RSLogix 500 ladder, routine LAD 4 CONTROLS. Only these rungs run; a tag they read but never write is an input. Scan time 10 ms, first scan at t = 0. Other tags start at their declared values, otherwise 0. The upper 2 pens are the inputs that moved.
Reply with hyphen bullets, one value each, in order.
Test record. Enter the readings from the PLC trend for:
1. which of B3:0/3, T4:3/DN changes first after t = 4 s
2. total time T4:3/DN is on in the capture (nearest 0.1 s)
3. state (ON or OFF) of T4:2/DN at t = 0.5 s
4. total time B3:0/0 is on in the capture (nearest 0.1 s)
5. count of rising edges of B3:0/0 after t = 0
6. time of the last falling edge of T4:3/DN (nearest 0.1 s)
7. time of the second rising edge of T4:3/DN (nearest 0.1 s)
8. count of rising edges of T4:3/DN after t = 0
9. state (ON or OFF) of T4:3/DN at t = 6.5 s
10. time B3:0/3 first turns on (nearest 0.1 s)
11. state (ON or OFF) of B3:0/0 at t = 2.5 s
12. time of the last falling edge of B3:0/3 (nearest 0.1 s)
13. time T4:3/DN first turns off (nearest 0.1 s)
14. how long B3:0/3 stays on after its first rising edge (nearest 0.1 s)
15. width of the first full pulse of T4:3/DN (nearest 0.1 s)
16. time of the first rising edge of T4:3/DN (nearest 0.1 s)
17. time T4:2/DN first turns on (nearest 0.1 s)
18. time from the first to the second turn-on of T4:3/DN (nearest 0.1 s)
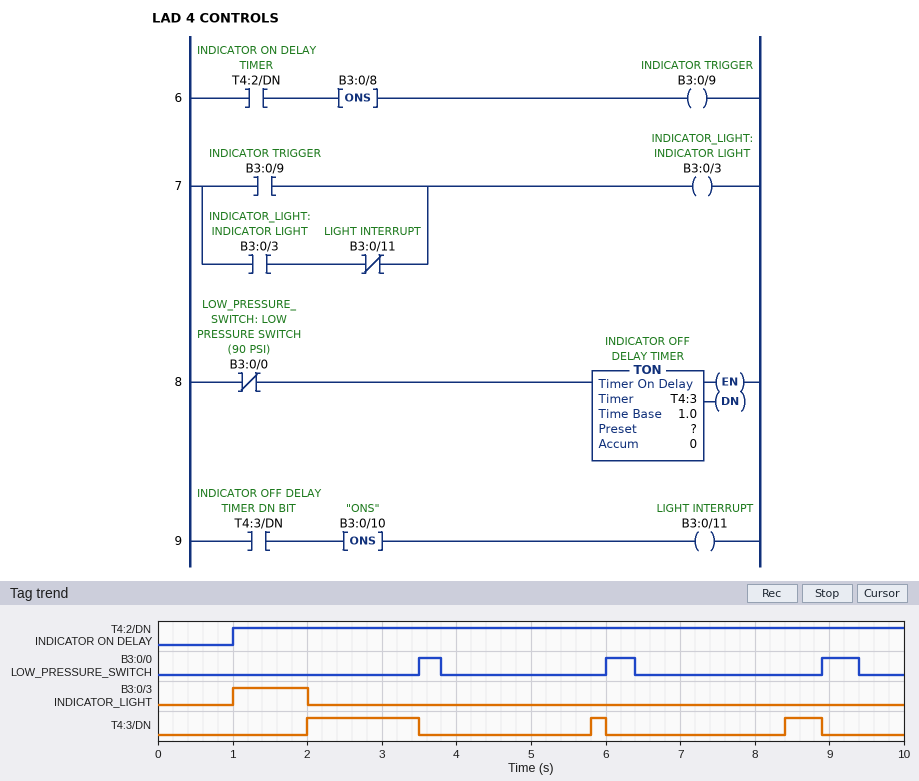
- T4:3/DN
- 2.2 s
- OFF
- 1.2 s
- 3
- 8.9 s
- 5.8 s
- 3
- OFF
- 1.0 s
- OFF
- 2.0 s
- 3.5 s
- 1.0 s
- 1.5 s
- 2.0 s
- 1.0 s
- 3.8 s
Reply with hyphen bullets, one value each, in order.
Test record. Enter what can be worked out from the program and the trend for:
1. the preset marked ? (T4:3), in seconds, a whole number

- 2 s
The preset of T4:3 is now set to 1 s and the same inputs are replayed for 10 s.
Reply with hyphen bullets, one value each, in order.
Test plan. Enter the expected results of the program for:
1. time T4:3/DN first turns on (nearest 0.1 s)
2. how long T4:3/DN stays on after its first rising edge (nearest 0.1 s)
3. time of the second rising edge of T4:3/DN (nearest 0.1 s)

- 1.0 s
- 2.5 s
- 4.8 s
